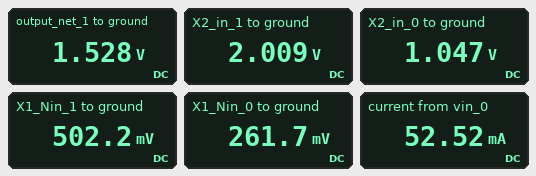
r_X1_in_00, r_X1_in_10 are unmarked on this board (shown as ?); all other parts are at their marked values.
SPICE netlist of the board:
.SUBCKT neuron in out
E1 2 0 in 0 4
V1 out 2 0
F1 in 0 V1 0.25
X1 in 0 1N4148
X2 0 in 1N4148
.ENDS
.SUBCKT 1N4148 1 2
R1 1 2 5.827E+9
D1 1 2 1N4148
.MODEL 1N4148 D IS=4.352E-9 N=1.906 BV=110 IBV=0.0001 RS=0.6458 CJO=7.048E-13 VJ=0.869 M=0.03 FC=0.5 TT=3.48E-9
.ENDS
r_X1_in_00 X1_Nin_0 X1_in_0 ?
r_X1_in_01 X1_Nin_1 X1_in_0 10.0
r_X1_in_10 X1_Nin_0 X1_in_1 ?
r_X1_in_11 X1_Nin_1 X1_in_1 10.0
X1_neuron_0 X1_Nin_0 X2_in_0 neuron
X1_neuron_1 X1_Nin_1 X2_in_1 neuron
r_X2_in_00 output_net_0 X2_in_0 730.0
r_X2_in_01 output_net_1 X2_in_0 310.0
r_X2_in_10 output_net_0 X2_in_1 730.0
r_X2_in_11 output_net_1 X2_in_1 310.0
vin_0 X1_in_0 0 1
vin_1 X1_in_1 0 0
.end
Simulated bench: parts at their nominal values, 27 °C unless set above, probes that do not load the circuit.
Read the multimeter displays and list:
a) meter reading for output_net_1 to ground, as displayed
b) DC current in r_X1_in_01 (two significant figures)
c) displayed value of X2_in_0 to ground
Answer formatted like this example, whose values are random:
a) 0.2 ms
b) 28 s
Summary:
a) 1.528 V
b) 50 mA
c) 1.047 V
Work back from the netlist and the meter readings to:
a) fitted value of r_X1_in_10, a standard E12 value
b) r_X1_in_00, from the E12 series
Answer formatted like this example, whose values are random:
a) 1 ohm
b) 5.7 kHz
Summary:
a) 120 Ω
b) 270 Ω
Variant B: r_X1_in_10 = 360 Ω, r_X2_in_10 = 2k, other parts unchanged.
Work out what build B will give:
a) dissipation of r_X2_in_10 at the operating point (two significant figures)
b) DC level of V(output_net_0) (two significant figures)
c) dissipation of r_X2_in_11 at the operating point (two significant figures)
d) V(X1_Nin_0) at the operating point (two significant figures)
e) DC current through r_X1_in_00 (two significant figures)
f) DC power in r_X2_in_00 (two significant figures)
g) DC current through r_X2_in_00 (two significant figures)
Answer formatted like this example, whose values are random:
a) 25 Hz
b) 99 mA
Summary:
a) 8.6 µW
b) 2.1 V
c) 26 µW
d) 540 mV
e) 1.7 mA
f) 3.1 µW
g) 66 µA
